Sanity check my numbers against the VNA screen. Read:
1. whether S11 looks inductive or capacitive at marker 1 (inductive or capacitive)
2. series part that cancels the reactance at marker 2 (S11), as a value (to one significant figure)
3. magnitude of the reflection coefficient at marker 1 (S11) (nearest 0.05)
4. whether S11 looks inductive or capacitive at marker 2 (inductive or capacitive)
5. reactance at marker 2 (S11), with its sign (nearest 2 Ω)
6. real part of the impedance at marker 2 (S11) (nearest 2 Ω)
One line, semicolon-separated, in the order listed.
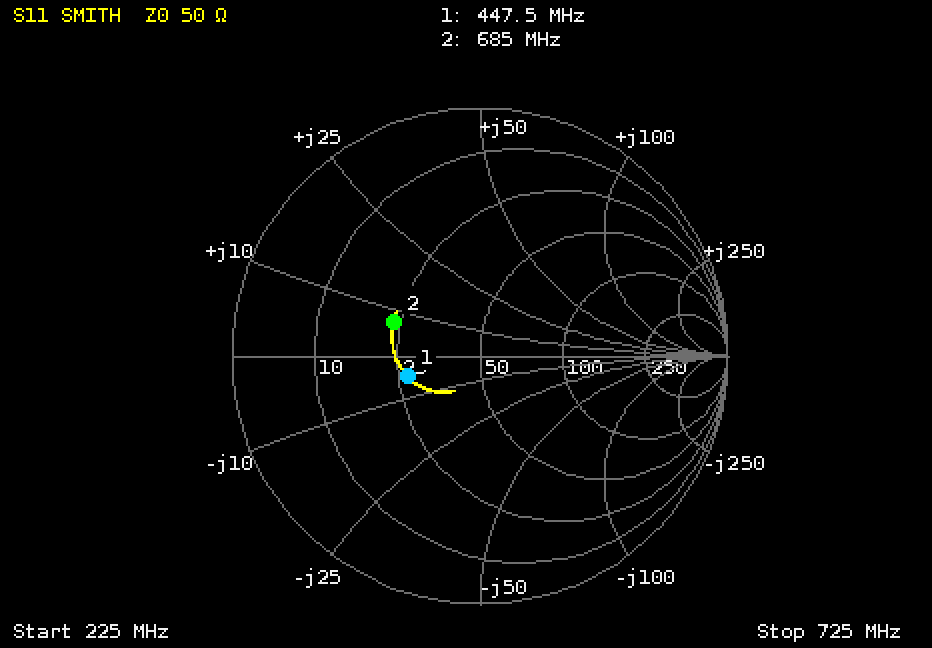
capacitive; 30 pF; 0.30; inductive; +8 Ω; 24 Ω
